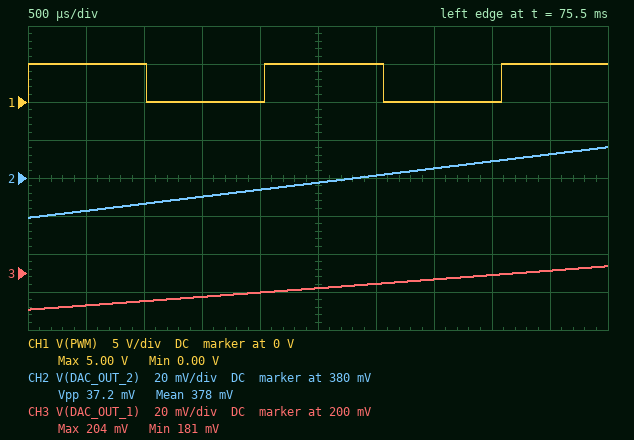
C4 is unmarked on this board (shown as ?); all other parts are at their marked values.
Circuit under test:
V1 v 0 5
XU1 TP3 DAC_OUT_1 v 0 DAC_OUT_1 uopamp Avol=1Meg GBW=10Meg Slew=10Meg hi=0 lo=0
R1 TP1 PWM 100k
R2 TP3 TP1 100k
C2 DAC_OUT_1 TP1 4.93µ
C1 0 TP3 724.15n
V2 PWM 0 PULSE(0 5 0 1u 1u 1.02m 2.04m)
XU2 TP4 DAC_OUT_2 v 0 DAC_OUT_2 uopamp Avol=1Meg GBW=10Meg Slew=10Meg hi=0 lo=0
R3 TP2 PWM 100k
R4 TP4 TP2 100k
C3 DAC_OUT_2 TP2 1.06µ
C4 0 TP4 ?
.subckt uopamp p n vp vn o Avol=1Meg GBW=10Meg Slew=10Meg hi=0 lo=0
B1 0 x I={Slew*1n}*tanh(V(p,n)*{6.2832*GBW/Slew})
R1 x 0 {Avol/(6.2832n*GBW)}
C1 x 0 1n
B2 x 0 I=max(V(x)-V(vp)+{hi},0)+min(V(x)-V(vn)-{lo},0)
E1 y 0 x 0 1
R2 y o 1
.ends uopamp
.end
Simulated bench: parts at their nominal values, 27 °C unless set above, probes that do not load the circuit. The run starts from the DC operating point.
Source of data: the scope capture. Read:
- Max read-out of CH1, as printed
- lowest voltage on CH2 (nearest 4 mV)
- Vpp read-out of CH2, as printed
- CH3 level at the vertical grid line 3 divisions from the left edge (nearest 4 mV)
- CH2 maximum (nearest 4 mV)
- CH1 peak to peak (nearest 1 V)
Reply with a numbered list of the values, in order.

1. 5.00 V
2. 360 mV
3. 37.2 mV
4. 188 mV
5. 396 mV
6. 5 V
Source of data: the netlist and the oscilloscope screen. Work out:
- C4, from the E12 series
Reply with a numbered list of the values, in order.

1. 1.2 µF
